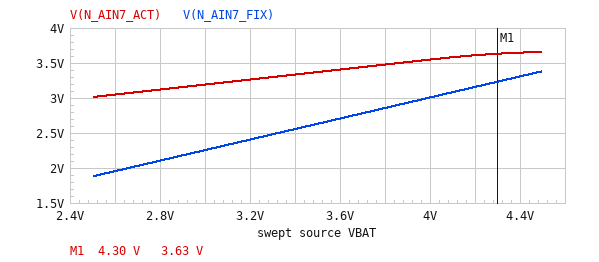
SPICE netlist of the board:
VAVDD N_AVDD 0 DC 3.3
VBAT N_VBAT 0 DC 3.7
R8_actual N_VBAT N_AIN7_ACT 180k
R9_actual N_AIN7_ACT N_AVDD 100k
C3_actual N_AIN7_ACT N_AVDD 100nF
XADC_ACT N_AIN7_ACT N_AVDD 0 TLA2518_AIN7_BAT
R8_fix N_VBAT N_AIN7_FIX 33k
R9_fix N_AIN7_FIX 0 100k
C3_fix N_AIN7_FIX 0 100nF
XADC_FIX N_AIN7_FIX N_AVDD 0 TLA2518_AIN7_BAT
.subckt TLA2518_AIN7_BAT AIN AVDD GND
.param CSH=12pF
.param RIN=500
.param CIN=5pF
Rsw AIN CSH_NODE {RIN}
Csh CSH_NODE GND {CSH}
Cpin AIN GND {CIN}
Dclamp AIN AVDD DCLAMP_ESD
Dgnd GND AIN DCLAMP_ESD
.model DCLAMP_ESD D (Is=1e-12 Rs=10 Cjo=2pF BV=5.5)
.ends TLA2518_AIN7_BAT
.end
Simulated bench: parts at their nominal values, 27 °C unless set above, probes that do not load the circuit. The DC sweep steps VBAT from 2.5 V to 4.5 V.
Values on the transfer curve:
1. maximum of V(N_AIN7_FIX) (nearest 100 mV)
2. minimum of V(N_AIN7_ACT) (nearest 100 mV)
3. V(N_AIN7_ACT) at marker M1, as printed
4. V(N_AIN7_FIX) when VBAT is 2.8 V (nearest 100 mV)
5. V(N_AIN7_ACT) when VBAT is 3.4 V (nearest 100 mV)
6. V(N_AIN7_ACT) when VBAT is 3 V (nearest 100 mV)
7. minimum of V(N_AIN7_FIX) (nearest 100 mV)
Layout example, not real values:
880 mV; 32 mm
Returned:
3.4 V; 3.0 V; 3.63 V; 2.1 V; 3.3 V; 3.2 V; 1.9 V
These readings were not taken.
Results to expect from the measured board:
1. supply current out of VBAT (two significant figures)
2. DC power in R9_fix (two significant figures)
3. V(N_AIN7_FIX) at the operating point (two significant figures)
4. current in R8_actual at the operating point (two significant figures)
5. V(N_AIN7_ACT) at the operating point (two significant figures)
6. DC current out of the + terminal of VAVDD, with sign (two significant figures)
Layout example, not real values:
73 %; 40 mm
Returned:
29 µA; 77 µW; 2.8 V; 1.4 µA; 3.4 V; -1.4 µA
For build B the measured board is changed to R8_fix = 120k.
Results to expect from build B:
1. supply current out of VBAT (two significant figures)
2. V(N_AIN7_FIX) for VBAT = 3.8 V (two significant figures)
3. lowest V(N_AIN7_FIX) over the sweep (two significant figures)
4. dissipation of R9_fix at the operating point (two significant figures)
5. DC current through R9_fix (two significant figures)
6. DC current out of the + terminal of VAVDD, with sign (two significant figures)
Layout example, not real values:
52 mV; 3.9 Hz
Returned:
18 µA; 1.7 V; 1.1 V; 28 µW; 17 µA; -1.4 µA
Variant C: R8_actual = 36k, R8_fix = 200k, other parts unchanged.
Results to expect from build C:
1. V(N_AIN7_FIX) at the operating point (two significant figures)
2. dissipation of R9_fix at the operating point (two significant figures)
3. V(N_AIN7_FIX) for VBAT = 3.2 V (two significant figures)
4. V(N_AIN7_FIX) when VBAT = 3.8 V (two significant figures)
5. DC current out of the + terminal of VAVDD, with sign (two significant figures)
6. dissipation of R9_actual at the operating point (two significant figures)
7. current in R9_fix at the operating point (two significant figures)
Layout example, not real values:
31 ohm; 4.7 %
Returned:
1.2 V; 15 µW; 1.1 V; 1.3 V; -3.0 µA; 850 nW; 12 µA
